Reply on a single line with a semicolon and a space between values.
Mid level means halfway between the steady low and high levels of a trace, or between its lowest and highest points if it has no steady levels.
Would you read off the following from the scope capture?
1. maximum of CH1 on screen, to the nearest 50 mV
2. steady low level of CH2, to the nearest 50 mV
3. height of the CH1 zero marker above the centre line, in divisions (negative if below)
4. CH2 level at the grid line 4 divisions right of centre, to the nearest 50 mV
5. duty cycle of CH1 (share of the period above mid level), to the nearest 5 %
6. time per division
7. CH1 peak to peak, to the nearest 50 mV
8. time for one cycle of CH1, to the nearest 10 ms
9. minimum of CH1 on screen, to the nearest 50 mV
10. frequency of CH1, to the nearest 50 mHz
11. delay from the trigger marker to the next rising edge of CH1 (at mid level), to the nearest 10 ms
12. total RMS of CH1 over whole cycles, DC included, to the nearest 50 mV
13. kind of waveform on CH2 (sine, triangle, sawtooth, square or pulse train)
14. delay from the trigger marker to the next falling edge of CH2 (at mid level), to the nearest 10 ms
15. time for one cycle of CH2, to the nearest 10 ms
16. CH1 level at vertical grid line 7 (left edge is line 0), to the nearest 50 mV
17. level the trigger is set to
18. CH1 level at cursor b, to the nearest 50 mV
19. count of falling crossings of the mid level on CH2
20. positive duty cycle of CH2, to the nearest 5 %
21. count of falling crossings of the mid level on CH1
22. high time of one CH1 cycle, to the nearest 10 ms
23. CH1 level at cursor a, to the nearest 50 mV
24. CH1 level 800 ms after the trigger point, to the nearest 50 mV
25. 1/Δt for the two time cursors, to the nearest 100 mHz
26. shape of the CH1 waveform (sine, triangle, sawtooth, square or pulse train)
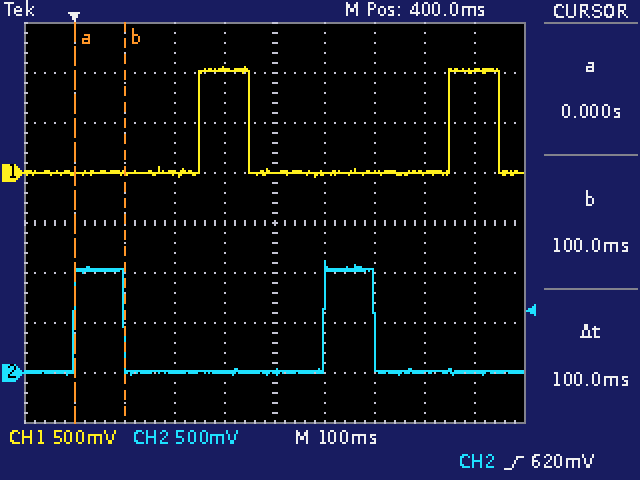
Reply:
1.05 V; 0 mV; +1.0 div; 0 mV; 20 %; 100 ms; 1.10 V; 500 ms; -50 mV; 2.00 Hz; 250 ms; 450 mV; pulse train; 100 ms; 500 ms; 0 mV; 620 mV; 0 mV; 2; 20 %; 2; 100 ms; 0 mV; 1.00 V; 10.0 Hz; pulse train
